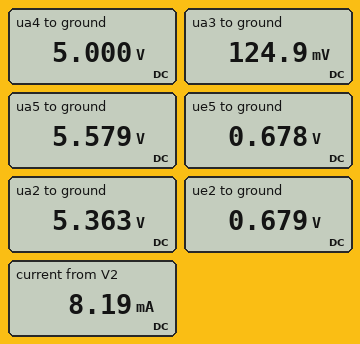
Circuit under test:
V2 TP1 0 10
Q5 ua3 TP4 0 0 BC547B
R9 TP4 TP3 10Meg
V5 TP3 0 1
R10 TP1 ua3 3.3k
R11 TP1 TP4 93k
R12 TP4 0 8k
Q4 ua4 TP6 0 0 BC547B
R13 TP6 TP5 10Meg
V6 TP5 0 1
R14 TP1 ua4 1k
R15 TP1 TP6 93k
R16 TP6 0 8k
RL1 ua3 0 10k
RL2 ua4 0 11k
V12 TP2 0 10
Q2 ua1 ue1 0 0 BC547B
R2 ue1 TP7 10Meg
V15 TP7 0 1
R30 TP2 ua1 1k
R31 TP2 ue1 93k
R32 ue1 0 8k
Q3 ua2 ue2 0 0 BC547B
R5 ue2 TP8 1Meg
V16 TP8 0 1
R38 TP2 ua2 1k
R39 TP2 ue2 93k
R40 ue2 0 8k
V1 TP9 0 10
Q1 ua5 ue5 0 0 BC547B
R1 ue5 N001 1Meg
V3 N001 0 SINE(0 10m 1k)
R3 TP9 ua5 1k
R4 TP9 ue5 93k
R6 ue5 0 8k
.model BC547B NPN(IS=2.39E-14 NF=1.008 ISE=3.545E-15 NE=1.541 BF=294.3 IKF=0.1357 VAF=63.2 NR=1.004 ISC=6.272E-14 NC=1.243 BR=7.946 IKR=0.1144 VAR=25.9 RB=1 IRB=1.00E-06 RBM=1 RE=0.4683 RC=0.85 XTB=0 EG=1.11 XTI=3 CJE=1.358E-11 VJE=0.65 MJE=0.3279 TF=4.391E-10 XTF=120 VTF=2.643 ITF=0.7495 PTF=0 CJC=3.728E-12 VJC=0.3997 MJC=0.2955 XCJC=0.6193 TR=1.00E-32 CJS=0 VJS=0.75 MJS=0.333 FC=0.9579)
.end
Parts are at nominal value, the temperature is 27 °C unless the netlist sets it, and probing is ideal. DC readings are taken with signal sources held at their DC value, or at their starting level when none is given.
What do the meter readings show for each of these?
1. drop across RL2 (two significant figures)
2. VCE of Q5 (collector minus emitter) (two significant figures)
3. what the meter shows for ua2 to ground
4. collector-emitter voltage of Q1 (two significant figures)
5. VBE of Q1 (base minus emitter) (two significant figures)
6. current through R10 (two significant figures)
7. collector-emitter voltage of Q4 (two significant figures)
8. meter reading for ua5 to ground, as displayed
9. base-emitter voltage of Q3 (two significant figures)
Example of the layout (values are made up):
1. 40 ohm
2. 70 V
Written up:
1. 5.0 V
2. 120 mV
3. 5.363 V
4. 5.6 V
5. 680 mV
6. 3.0 mA
7. 5.0 V
8. 5.579 V
9. 680 mV
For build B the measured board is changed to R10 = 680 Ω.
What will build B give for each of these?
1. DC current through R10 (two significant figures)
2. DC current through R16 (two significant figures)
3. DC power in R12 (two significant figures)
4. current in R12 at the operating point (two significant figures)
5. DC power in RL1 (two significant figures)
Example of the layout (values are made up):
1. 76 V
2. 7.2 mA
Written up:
1. 5.3 mA
2. 85 µA
3. 58 µW
4. 85 µA
5. 4.1 mW
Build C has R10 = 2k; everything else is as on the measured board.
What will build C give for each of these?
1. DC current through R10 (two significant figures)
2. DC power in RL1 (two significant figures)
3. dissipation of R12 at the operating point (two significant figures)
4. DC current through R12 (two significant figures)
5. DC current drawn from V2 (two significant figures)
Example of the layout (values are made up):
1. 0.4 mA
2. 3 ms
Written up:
1. 4.4 mA
2. 140 µW
3. 58 µW
4. 85 µA
5. 9.6 mA
